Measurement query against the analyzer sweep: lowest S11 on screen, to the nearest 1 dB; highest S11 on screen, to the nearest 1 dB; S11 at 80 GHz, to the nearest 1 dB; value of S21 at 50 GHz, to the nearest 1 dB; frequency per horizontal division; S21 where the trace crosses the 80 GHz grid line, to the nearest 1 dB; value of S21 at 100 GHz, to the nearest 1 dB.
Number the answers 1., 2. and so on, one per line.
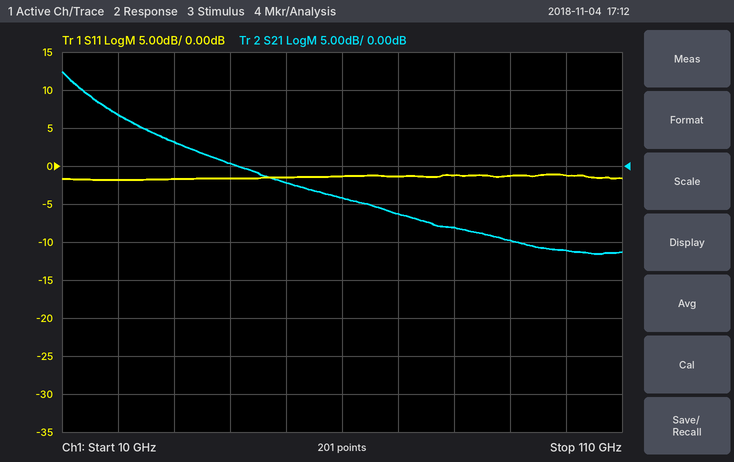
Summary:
1. -2 dB
2. -1 dB
3. -1 dB
4. -2 dB
5. 10 GHz
6. -8 dB
7. -11 dB
